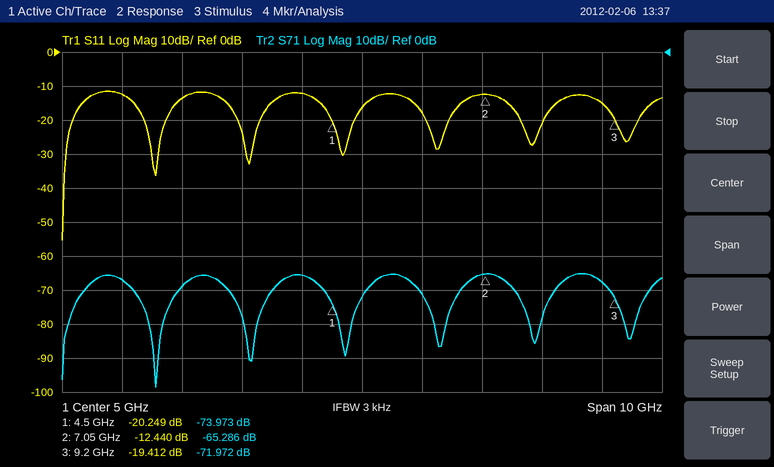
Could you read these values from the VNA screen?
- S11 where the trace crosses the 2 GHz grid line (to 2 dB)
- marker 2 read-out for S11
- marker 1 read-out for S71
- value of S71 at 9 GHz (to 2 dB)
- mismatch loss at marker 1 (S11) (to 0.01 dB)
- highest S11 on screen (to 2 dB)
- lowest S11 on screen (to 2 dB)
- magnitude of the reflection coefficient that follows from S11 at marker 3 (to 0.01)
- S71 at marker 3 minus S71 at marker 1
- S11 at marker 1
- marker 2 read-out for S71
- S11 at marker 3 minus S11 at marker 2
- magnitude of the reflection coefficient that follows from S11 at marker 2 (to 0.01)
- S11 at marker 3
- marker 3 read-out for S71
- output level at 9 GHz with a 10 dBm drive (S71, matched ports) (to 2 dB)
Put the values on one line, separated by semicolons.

-14 dB; -12.440 dB; -73.973 dB; -68 dB; 0.04 dB; -12 dB; -56 dB; 0.11; 2.001 dB; -20.249 dB; -65.286 dB; -6.972 dB; 0.24; -19.412 dB; -71.972 dB; -58 dBm
